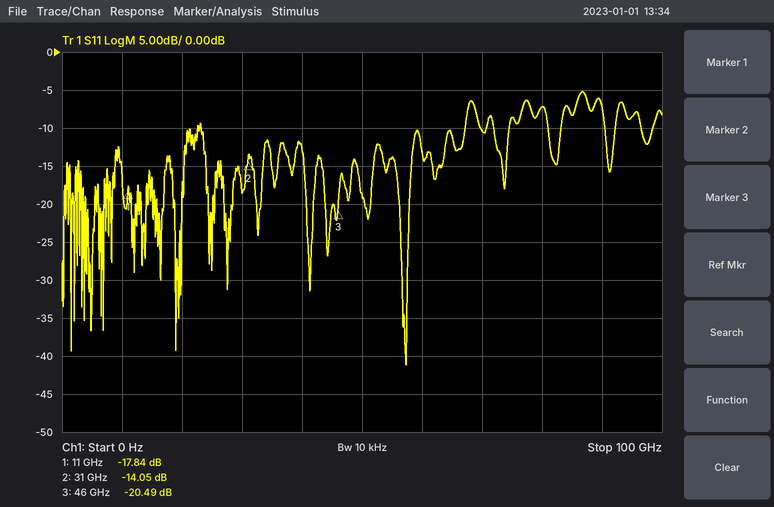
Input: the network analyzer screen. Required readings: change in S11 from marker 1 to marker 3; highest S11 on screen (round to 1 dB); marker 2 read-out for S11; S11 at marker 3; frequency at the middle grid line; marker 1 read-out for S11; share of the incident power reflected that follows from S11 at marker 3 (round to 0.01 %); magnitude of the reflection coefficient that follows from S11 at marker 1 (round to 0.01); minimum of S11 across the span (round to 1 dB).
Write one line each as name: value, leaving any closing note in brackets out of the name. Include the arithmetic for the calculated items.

change in S11 from marker 1 to marker 3: -20.49 − (-17.84) = -2.65 dB
highest S11 on screen: -5 dB
marker 2 read-out for S11: -14.05 dB
S11 at marker 3: -20.49 dB
frequency at the middle grid line: 50 GHz
marker 1 read-out for S11: -17.84 dB
share of the incident power reflected that follows from S11 at marker 3: 10^(-20.49/10) ≈ 0.89 %
magnitude of the reflection coefficient that follows from S11 at marker 1: 10^(-17.84/20) ≈ 0.13
minimum of S11 across the span: -41 dB
